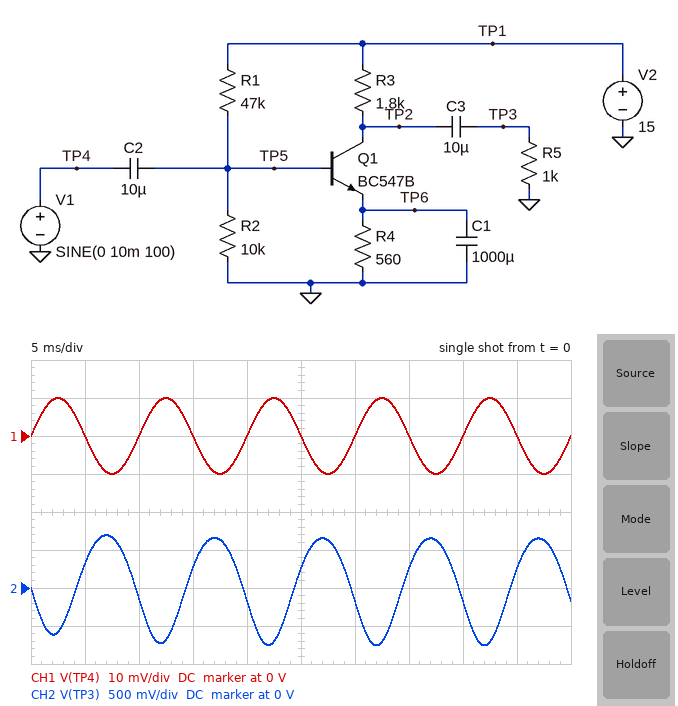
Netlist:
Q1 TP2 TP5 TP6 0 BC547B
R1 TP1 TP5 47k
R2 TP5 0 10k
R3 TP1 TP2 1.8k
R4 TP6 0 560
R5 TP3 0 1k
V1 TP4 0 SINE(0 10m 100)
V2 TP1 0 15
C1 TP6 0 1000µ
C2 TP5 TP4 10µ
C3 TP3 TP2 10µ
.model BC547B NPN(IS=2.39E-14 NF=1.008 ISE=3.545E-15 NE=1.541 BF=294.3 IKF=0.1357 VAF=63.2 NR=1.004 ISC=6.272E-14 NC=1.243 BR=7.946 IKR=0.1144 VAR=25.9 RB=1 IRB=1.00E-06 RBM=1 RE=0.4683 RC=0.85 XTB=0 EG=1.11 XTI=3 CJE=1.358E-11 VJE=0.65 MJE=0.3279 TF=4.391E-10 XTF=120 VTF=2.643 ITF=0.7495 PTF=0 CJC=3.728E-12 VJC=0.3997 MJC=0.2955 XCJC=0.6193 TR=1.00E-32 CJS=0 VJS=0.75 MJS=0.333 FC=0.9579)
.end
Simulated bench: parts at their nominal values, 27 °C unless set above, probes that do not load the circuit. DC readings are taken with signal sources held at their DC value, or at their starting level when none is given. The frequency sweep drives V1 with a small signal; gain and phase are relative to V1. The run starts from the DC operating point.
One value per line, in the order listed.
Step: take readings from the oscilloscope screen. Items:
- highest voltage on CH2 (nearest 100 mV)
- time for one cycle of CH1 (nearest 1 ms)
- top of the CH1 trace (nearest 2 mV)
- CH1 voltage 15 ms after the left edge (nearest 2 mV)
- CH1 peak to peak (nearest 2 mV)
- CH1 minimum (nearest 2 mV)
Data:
700 mV
10 ms
10 mV
0 V
20 mV
-10 mV
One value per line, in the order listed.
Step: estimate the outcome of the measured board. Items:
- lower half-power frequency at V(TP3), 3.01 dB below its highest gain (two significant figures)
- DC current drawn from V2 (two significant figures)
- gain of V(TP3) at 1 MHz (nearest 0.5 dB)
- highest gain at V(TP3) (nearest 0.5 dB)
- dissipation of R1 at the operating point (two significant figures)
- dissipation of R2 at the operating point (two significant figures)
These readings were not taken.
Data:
27 Hz
3.6 mA
37.5 dB
37.5 dB
3.3 mW
650 µW
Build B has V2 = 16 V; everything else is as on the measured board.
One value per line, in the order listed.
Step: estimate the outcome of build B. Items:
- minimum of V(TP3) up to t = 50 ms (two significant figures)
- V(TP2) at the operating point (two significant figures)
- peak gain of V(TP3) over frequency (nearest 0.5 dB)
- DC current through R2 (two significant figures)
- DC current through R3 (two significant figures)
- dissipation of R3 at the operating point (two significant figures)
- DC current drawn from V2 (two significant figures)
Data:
-810 mV
9.5 V
38.0 dB
270 µA
3.6 mA
24 mW
3.9 mA
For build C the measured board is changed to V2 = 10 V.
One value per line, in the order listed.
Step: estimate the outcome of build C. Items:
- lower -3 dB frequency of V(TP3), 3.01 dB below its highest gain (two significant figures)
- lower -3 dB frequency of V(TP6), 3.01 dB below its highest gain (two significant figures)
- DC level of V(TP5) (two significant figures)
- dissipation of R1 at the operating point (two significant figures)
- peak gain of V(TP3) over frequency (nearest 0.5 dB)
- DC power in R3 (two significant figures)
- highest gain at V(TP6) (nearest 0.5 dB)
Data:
17 Hz
1.2 Hz
1.7 V
1.5 mW
32.5 dB
6.3 mW
-4.0 dB
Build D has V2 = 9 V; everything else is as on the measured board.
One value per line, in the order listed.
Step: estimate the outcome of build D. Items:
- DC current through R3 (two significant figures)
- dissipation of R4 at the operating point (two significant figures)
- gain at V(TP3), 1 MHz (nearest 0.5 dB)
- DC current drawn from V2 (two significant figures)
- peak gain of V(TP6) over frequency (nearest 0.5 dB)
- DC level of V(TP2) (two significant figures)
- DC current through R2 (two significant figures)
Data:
1.6 mA
1.4 mW
31.5 dB
1.7 mA
-4.0 dB
6.2 V
150 µA
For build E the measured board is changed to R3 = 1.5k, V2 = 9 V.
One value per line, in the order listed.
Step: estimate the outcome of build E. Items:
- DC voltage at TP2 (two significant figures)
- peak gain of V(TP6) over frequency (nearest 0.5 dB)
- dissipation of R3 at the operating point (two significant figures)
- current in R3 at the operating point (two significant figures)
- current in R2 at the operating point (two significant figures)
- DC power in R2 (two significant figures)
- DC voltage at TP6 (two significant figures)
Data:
6.6 V
-4.0 dB
3.7 mW
1.6 mA
150 µA
240 µW
890 mV
